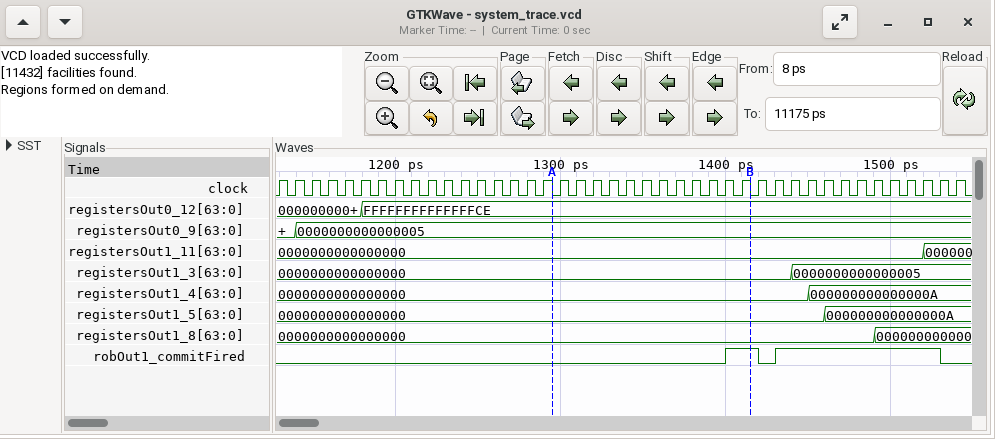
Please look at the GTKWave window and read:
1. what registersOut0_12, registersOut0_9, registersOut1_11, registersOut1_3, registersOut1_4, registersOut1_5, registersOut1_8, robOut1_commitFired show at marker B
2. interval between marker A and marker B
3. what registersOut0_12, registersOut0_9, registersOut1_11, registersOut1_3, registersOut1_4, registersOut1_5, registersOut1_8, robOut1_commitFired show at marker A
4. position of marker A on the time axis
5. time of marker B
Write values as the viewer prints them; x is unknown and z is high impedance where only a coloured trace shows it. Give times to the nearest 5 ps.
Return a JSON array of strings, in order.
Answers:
["registersOut0_12=FFFFFFFFFFFFFFCE, registersOut0_9=0000000000000005, registersOut1_11=0000000000000000, registersOut1_3=0000000000000000, registersOut1_4=0000000000000000, registersOut1_5=0000000000000000, registersOut1_8=0000000000000000, robOut1_commitFired=1", "120 ps", "registersOut0_12=FFFFFFFFFFFFFFCE, registersOut0_9=0000000000000005, registersOut1_11=0000000000000000, registersOut1_3=0000000000000000, registersOut1_4=0000000000000000, registersOut1_5=0000000000000000, registersOut1_8=0000000000000000, robOut1_commitFired=0", "1295 ps", "1415 ps"]
